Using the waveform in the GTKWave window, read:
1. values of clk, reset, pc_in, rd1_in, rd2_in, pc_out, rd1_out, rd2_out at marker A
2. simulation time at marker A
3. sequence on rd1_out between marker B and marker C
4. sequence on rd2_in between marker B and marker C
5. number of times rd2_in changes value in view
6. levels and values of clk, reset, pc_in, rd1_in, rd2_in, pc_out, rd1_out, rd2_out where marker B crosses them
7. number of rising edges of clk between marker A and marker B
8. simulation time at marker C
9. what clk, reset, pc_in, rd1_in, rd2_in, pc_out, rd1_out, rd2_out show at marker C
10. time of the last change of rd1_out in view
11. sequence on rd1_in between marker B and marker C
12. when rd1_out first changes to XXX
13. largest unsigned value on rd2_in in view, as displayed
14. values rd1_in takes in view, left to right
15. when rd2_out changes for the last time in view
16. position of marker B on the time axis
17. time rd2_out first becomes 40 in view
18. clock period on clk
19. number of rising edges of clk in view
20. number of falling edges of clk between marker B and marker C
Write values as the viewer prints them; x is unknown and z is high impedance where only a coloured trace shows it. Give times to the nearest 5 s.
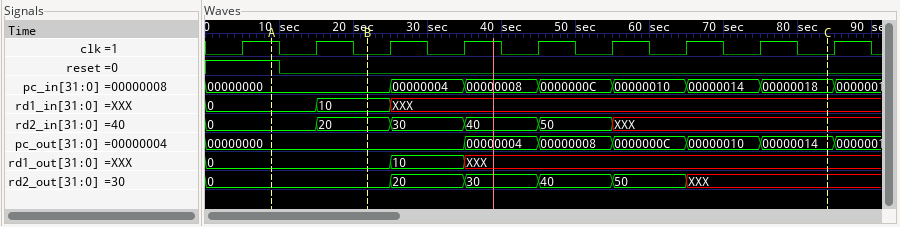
clk=1, reset=1, pc_in=00000000, rd1_in=0, rd2_in=0, pc_out=00000000, rd1_out=0, rd2_out=0
10 s
0, 10, XXX
20, 30, 40, 50, XXX
5
clk=0, reset=0, pc_in=00000000, rd1_in=10, rd2_in=20, pc_out=00000000, rd1_out=0, rd2_out=0
1
85 s
clk=0, reset=0, pc_in=00000018, rd1_in=XXX, rd2_in=XXX, pc_out=00000014, rd1_out=XXX, rd2_out=XXX
35 s
10, XXX
35 s
50
0, 10, XXX
65 s
20 s
45 s
10 s
9
6
